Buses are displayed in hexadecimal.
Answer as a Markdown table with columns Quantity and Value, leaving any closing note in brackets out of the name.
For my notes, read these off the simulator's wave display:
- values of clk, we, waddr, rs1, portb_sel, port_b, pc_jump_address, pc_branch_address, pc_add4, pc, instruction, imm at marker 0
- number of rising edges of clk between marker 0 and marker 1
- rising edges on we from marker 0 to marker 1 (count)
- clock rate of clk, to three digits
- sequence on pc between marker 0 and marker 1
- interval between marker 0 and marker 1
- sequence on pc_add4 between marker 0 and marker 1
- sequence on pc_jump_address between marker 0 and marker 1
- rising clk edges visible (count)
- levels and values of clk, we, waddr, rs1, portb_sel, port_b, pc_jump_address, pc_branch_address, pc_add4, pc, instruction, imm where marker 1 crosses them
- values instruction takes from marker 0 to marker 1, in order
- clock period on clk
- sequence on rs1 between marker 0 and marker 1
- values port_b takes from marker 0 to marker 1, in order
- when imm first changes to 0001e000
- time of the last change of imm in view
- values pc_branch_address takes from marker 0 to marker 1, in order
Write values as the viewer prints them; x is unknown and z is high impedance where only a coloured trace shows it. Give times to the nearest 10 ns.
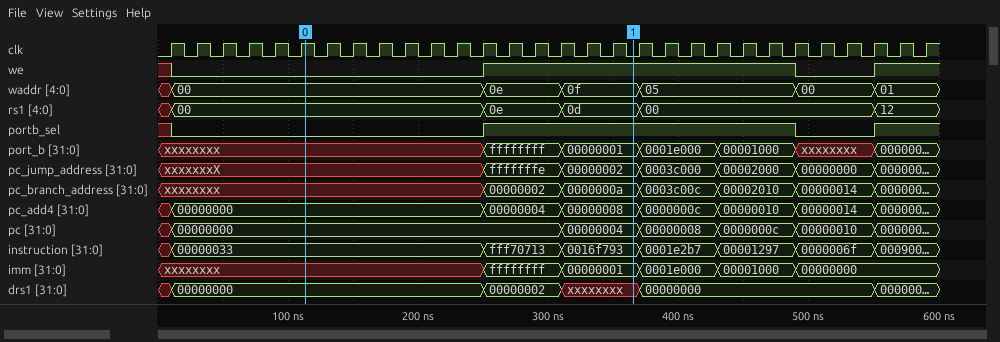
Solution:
| Quantity | Value |
|---|---|
| values of clk, we, waddr, rs1, portb_sel, port_b, pc_jump_address, pc_branch_address, pc_add4, pc, instruction, imm at marker 0 | clk=1, we=0, waddr=00, rs1=00, portb_sel=0, port_b=xxxxxxxx, pc_jump_address=xxxxxxxX, pc_branch_address=xxxxxxxx, pc_add4=00000000, pc=00000000, instruction=00000033, imm=xxxxxxxx |
| number of rising edges of clk between marker 0 and marker 1 | 12 |
| rising edges on we from marker 0 to marker 1 | 1 |
| clock rate of clk, to three digits | 50.0 MHz |
| sequence on pc between marker 0 and marker 1 | 00000000, 00000004 |
| interval between marker 0 and marker 1 | 250 ns |
| sequence on pc_add4 between marker 0 and marker 1 | 00000000, 00000004, 00000008 |
| sequence on pc_jump_address between marker 0 and marker 1 | xxxxxxxX, fffffffe, 00000002 |
| rising clk edges visible | 30 |
| levels and values of clk, we, waddr, rs1, portb_sel, port_b, pc_jump_address, pc_branch_address, pc_add4, pc, instruction, imm where marker 1 crosses them | clk=0, we=1, waddr=0f, rs1=0d, portb_sel=1, port_b=00000001, pc_jump_address=00000002, pc_branch_address=0000000a, pc_add4=00000008, pc=00000004, instruction=0016f793, imm=00000001 |
| values instruction takes from marker 0 to marker 1, in order | 00000033, fff70713, 0016f793 |
| clock period on clk | 20 ns |
| sequence on rs1 between marker 0 and marker 1 | 00, 0e, 0d |
| values port_b takes from marker 0 to marker 1, in order | xxxxxxxx, ffffffff, 00000001 |
| when imm first changes to 0001e000 | 370 ns |
| time of the last change of imm in view | 490 ns |
| values pc_branch_address takes from marker 0 to marker 1, in order | xxxxxxxx, 00000002, 0000000a |
